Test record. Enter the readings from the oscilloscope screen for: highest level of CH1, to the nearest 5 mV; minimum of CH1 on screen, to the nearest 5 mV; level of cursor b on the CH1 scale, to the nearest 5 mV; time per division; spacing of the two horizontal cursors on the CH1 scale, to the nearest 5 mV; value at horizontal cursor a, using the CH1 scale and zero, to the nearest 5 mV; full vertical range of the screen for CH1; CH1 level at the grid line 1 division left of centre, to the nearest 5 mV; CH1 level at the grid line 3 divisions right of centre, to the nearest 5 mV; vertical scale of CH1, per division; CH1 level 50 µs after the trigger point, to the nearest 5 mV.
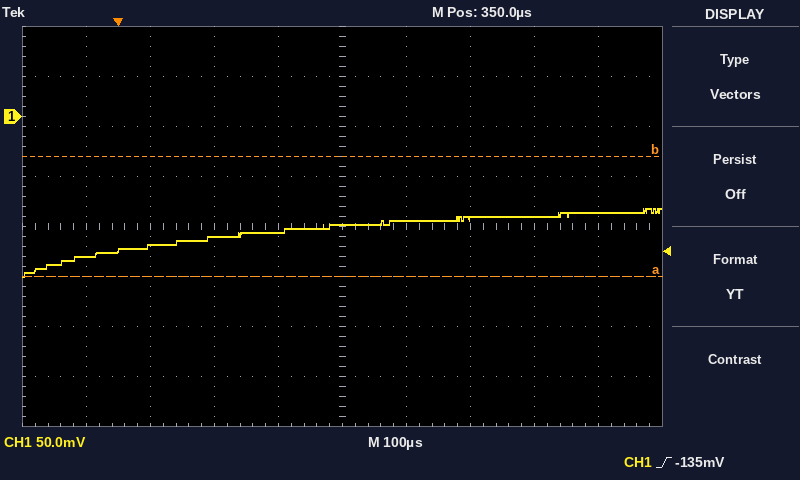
-90 mV
-160 mV
-40 mV
100 µs
120 mV
-160 mV
400 mV
-115 mV
-100 mV
50 mV
-130 mV
